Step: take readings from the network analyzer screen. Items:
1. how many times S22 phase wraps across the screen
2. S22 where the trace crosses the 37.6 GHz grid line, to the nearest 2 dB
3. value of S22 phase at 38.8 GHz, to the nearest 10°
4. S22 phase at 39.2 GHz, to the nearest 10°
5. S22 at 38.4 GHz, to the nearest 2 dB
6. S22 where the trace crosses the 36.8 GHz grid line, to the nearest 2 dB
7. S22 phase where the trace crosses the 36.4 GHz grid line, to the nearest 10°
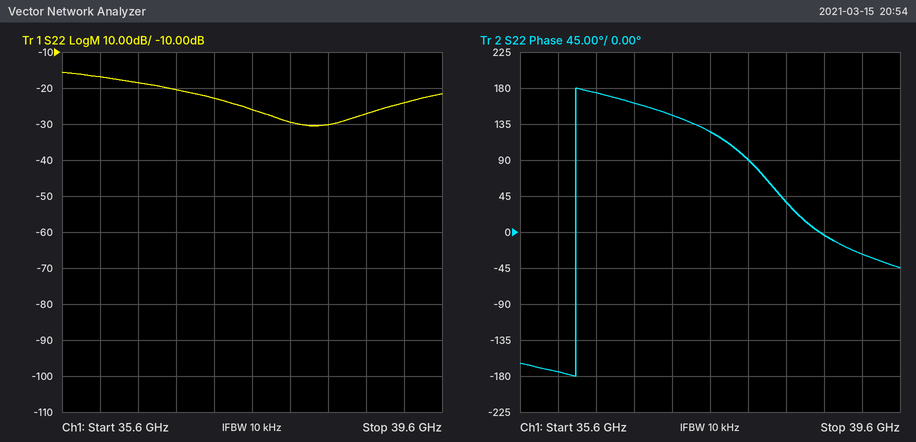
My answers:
1
-26 dB
0°
-30°
-30 dB
-20 dB
170°
